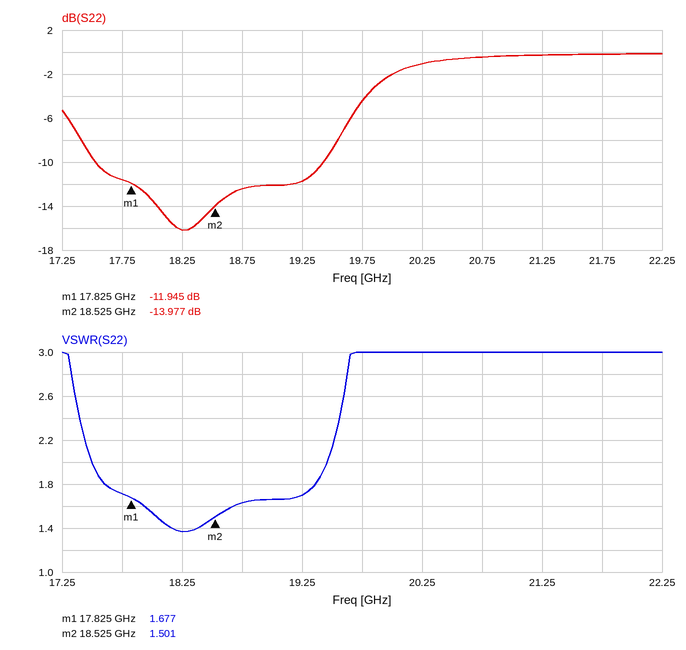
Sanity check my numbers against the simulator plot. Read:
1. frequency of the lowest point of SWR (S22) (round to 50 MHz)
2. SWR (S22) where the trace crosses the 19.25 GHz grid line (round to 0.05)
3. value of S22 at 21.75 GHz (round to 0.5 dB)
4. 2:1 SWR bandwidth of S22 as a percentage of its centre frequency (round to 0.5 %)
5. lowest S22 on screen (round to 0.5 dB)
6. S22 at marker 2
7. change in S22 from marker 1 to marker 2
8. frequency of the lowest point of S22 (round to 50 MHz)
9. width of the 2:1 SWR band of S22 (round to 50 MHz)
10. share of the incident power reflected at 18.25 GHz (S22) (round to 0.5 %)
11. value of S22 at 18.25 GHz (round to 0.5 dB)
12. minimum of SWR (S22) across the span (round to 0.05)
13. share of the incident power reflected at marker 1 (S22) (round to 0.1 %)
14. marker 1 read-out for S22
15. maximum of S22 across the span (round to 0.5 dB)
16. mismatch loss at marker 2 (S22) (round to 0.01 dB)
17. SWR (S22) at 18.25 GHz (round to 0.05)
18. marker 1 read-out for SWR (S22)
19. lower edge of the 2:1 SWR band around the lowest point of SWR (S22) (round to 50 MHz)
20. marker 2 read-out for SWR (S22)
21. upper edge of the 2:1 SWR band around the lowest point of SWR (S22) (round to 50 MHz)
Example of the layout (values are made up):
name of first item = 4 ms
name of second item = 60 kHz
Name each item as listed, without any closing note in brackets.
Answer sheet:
frequency of the lowest point of SWR (S22) = 18.25 GHz
SWR (S22) where the trace crosses the 19.25 GHz grid line = 1.70
value of S22 at 21.75 GHz = 0.0 dB
2:1 SWR bandwidth of S22 as a percentage of its centre frequency = 10.5 %
lowest S22 on screen = -16.0 dB
S22 at marker 2 = -13.977 dB
change in S22 from marker 1 to marker 2 = -2.032 dB
frequency of the lowest point of S22 = 18.25 GHz
width of the 2:1 SWR band of S22 = 1.95 GHz
share of the incident power reflected at 18.25 GHz (S22) = 2.5 %
value of S22 at 18.25 GHz = -16.0 dB
minimum of SWR (S22) across the span = 1.35
share of the incident power reflected at marker 1 (S22) = 6.4 %
marker 1 read-out for S22 = -11.945 dB
maximum of S22 across the span = 0.0 dB
mismatch loss at marker 2 (S22) = 0.18 dB
SWR (S22) at 18.25 GHz = 1.35
marker 1 read-out for SWR = 1.677
lower edge of the 2:1 SWR band around the lowest point of SWR (S22) = 17.50 GHz
marker 2 read-out for SWR = 1.501
upper edge of the 2:1 SWR band around the lowest point of SWR (S22) = 19.45 GHz
